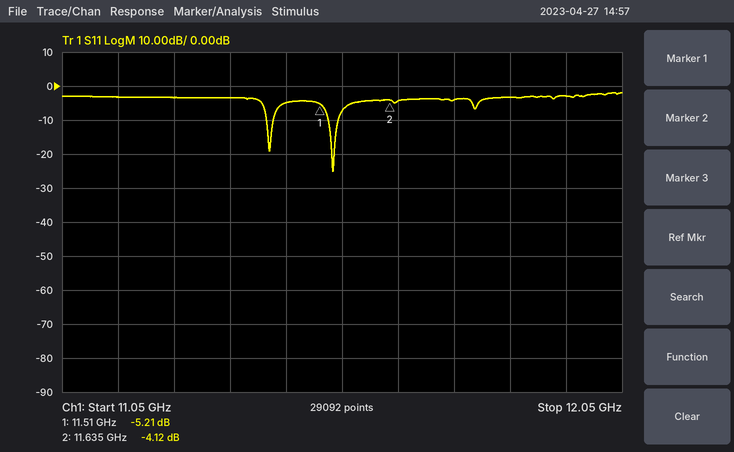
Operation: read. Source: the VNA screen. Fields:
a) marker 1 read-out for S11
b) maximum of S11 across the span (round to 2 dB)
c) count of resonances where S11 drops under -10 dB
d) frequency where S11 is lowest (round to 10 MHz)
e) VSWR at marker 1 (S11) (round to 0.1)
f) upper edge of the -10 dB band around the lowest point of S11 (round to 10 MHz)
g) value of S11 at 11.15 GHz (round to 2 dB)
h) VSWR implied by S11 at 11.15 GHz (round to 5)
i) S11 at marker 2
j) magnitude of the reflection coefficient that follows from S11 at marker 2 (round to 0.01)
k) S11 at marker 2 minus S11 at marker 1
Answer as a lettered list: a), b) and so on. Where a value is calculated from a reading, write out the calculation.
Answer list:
a) -5.21 dB
b) -2 dB
c) 2
d) 11.53 GHz
e) (1 + 0.5489)/(1 − 0.5489) ≈ 3.4
f) 11.54 GHz
g) -4 dB
h) |Γ| = 10^(-4/20) = 0.6310; VSWR = (1 + 0.6310)/(1 − 0.6310) ≈ 4.42, so 5 to the nearest 5
i) -4.12 dB
j) 10^(-4.12/20) ≈ 0.62
k) -4.12 − (-5.21) = 1.09 dB
